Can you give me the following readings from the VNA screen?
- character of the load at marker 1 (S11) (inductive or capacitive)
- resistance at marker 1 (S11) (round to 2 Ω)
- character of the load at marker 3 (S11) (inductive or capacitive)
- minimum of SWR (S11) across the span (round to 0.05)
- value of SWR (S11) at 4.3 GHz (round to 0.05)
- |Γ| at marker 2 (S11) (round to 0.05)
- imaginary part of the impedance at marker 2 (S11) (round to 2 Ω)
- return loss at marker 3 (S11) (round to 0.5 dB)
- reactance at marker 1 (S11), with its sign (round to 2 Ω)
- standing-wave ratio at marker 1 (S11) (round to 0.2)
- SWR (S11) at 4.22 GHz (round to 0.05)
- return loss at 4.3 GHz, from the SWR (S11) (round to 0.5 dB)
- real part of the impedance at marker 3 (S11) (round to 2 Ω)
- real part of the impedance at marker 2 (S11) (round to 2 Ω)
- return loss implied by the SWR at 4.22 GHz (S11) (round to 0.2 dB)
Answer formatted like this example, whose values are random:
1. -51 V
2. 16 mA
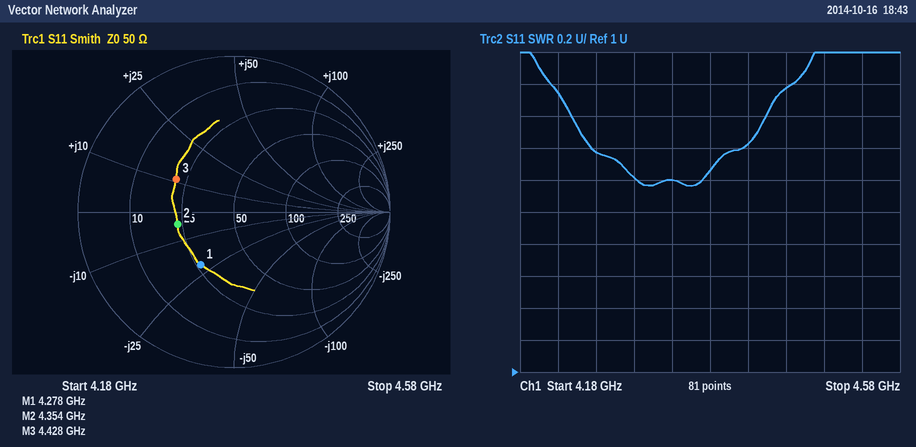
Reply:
1. capacitive
2. 26 Ω
3. inductive
4. 2.15
5. 2.20
6. 0.35
7. -4 Ω
8. 7.5 dB
9. -22 Ω
10. 2.4
11. 2.75
12. 8.5 dB
13. 22 Ω
14. 24 Ω
15. 6.6 dB
